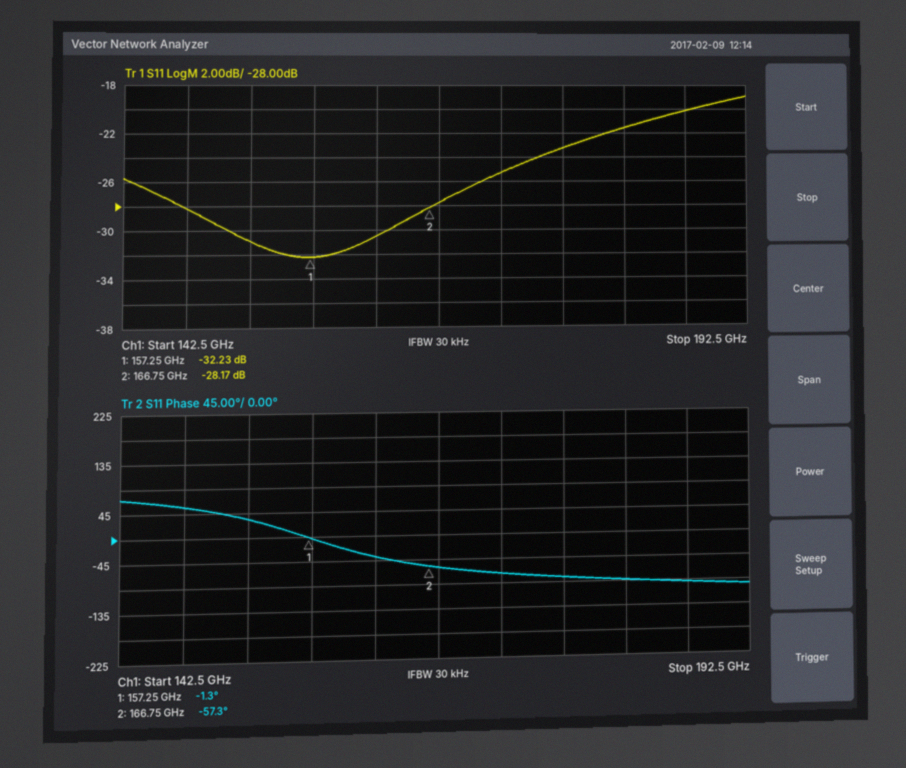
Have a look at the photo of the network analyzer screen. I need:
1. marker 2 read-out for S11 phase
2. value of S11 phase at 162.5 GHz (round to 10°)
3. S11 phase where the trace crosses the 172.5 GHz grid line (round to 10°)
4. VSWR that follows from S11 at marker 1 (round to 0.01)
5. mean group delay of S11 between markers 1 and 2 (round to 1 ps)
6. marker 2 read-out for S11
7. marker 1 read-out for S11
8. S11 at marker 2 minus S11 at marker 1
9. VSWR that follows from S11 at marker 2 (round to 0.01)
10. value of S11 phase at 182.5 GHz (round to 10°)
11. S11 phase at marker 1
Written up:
-57.3°
-40°
-70°
1.05
16 ps
-28.17 dB
-32.23 dB
4.06 dB
1.08
-90°
-1.3°
